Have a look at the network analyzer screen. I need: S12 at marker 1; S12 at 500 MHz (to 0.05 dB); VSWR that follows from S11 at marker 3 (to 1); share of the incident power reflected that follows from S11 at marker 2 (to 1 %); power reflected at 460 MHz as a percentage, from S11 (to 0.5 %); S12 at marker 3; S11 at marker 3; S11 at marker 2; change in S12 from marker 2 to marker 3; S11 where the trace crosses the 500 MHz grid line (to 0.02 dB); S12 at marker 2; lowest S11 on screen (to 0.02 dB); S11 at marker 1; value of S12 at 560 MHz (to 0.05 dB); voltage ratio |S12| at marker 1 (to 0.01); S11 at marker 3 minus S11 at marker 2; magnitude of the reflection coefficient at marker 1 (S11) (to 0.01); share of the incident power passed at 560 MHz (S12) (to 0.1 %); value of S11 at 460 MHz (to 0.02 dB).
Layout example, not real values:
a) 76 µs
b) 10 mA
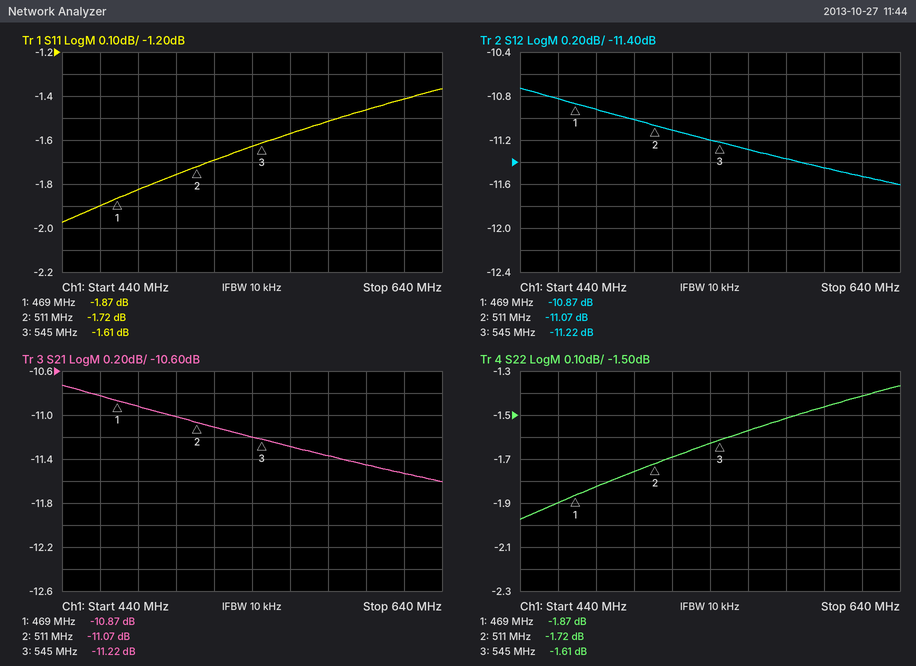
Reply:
a) -10.87 dB
b) -11.00 dB
c) 11
d) 67 %
e) 64.5 %
f) -11.22 dB
g) -1.61 dB
h) -1.72 dB
i) -0.15 dB
j) -1.76 dB
k) -11.07 dB
l) -1.98 dB
m) -1.87 dB
n) -11.30 dB
o) 0.29
p) 0.11 dB
q) 0.81
r) 7.4 %
s) -1.90 dB
